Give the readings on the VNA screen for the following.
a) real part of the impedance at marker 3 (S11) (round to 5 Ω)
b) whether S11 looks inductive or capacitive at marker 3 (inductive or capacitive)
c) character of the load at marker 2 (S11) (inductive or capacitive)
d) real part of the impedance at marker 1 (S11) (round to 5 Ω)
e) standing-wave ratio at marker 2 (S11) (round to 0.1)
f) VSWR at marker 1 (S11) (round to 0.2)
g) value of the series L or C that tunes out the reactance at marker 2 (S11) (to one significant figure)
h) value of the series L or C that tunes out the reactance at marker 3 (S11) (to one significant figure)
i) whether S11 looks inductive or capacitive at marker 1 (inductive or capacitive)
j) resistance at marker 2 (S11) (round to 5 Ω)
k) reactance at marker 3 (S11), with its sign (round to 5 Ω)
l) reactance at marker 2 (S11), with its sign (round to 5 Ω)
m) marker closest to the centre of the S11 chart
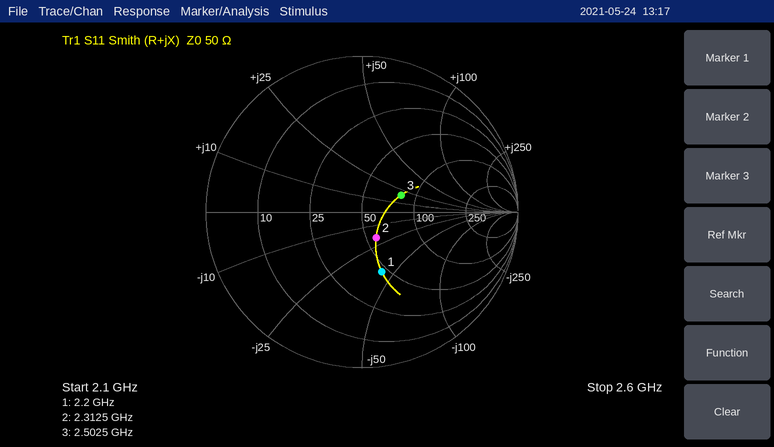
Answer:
80 Ω
inductive
capacitive
45 Ω
1.5
2.4
1 nH
3 pF
capacitive
55 Ω
+20 Ω
-20 Ω
marker 2
